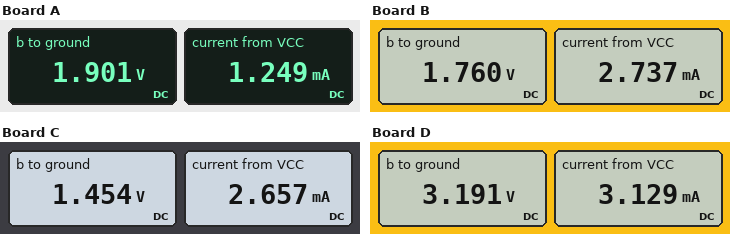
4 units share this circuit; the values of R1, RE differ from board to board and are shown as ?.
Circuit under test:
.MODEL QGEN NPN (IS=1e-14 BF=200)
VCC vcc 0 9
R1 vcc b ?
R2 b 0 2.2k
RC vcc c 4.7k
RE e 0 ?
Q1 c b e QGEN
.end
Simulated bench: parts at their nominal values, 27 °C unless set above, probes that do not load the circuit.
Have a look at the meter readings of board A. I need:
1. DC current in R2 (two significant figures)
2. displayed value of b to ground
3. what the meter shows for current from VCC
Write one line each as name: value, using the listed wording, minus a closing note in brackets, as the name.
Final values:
DC current in R2: 860 µA
displayed value of b to ground: 1.901 V
what the meter shows for current from VCC: 1.249 mA
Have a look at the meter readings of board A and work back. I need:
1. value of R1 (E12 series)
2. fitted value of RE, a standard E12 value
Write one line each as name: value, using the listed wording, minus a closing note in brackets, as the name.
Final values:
value of R1: 8.2 kΩ
fitted value of RE, a standard E12 value: 3.3 kΩ
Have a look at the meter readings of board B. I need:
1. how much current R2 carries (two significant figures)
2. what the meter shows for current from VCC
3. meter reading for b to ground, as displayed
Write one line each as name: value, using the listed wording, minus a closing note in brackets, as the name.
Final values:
how much current R2 carries: 800 µA
what the meter shows for current from VCC: 2.737 mA
meter reading for b to ground, as displayed: 1.760 V
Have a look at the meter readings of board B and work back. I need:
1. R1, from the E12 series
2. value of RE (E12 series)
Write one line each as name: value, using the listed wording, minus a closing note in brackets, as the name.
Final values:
R1, from the E12 series: 6.8 kΩ
value of RE: 560 Ω
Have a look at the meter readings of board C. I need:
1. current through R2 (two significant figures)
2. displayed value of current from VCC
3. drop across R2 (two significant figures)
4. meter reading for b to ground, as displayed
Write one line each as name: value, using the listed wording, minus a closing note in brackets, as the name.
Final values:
current through R2: 660 µA
displayed value of current from VCC: 2.657 mA
drop across R2: 1.5 V
meter reading for b to ground, as displayed: 1.454 V
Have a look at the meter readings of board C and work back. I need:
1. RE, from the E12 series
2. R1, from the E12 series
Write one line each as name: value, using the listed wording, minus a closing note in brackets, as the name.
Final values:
RE, from the E12 series: 390 Ω
R1, from the E12 series: 8.2 kΩ
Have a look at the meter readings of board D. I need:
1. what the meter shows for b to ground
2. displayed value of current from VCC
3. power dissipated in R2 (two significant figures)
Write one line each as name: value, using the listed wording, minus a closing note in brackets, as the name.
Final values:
what the meter shows for b to ground: 3.191 V
displayed value of current from VCC: 3.129 mA
power dissipated in R2: 4.6 mW
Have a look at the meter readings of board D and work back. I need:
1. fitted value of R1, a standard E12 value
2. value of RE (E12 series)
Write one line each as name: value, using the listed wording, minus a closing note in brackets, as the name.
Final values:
fitted value of R1, a standard E12 value: 3.3 kΩ
value of RE: 1.5 kΩ
